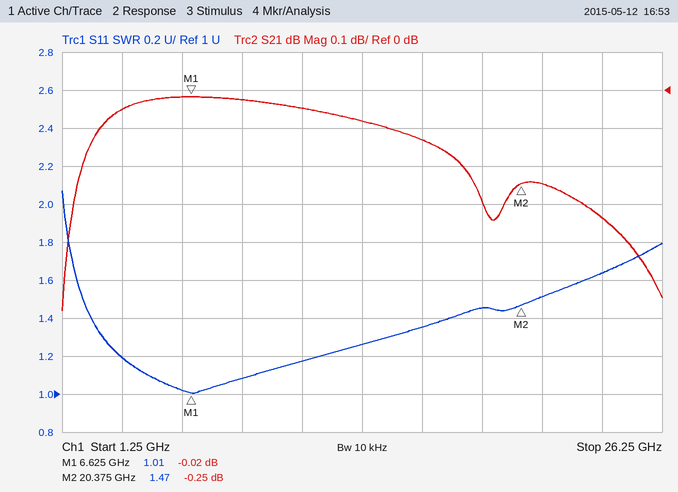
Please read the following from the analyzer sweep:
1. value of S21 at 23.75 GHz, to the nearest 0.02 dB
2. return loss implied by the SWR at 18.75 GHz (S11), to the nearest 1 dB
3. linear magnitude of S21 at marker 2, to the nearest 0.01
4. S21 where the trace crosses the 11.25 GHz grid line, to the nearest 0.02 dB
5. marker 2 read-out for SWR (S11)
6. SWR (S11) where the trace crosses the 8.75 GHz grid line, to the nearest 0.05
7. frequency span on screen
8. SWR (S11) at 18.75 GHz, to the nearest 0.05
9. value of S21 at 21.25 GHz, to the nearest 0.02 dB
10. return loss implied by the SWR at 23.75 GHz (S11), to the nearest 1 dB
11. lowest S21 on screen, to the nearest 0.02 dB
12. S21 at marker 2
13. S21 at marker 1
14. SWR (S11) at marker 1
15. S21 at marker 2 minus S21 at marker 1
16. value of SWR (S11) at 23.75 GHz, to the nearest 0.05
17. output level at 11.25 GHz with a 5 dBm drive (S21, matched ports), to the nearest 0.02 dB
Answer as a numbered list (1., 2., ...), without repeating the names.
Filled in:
1. -0.34 dB
2. 15 dB
3. 0.97
4. -0.04 dB
5. 1.47
6. 1.10
7. 25 GHz
8. 1.45
9. -0.24 dB
10. 12 dB
11. -0.58 dB
12. -0.25 dB
13. -0.02 dB
14. 1.01
15. -0.23 dB
16. 1.65
17. 4.96 dBm
